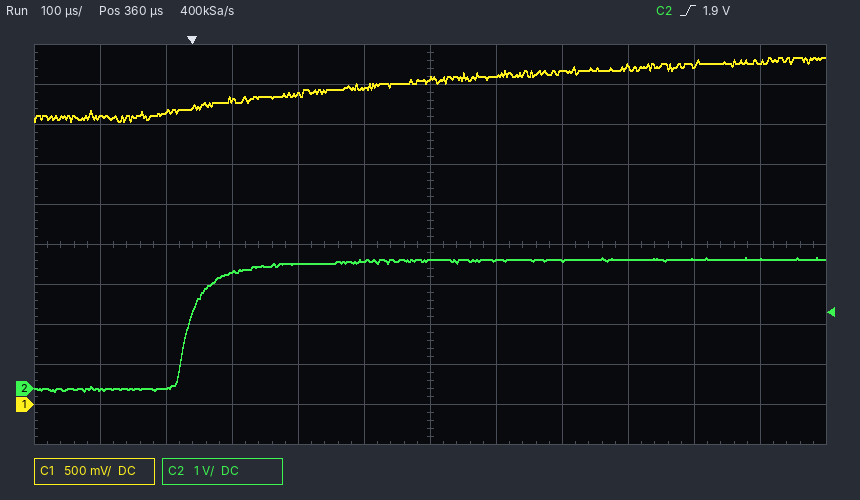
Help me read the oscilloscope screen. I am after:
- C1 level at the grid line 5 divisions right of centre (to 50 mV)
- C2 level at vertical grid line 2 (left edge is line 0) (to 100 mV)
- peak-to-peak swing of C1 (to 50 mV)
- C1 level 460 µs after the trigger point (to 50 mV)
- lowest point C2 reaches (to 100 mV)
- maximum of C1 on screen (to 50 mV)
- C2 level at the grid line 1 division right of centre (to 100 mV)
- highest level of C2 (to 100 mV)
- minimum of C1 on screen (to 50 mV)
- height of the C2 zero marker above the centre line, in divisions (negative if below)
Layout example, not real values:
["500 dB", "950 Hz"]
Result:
["4.30 V", "0.0 V", "800 mV", "4.10 V", "-100 mV", "4.35 V", "3.2 V", "3.3 V", "3.55 V", "-3.6 div"]
